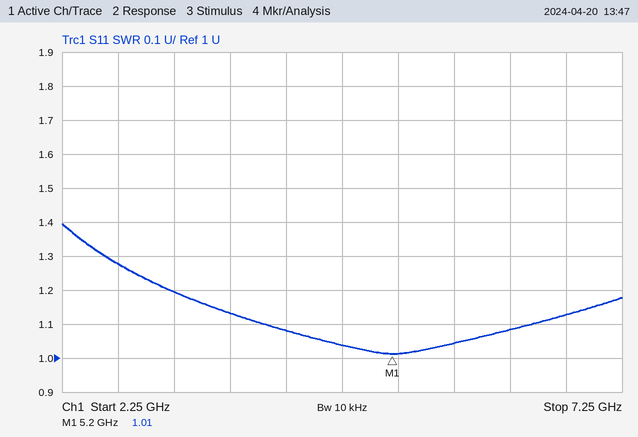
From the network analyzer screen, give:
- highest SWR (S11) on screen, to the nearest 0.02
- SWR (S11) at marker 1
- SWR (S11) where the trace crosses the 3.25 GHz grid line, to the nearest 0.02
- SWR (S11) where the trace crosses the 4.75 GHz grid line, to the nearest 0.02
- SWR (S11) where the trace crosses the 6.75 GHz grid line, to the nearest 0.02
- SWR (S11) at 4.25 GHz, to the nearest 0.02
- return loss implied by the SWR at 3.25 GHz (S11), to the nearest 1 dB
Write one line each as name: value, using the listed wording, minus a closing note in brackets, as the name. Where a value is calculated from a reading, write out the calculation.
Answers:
highest SWR (S11) on screen, to the nearest 0.02: 1.40
SWR (S11) at marker 1: 1.01
SWR (S11) where the trace crosses the 3.25 GHz grid line, to the nearest 0.02: 1.20
SWR (S11) where the trace crosses the 4.75 GHz grid line, to the nearest 0.02: 1.04
SWR (S11) where the trace crosses the 6.75 GHz grid line, to the nearest 0.02: 1.12
SWR (S11) at 4.25 GHz, to the nearest 0.02: 1.08
return loss implied by the SWR at 3.25 GHz (S11), to the nearest 1 dB: −20 log10((1.2 − 1)/(1.2 + 1)) ≈ 21 dB
